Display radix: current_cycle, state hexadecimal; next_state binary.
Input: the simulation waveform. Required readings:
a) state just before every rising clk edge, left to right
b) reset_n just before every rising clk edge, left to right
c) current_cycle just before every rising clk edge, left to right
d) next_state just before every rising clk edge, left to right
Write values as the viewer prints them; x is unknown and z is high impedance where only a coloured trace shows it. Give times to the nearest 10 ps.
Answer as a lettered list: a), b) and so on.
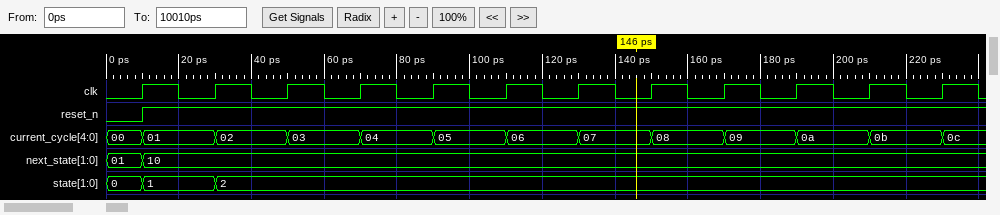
a) 0, 1, 2, 2, 2, 2, 2, 2, 2, 2, 2, 2
b) 0 1 1 1 1 1 1 1 1 1 1 1
c) 00, 01, 02, 03, 04, 05, 06, 07, 08, 09, 0a, 0b
d) 01, 10, 10, 10, 10, 10, 10, 10, 10, 10, 10, 10
